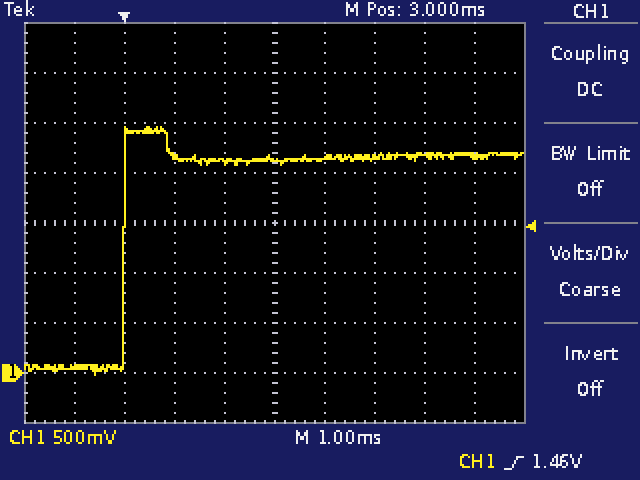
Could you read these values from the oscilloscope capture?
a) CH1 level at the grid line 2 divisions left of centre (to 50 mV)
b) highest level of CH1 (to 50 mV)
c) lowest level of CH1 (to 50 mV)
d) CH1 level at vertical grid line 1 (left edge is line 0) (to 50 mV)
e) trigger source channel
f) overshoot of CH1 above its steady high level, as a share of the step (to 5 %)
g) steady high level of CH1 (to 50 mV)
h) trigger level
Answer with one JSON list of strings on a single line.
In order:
["2.15 V", "2.45 V", "0 mV", "50 mV", "CH1", "15 %", "2.15 V", "1.46 V"]
